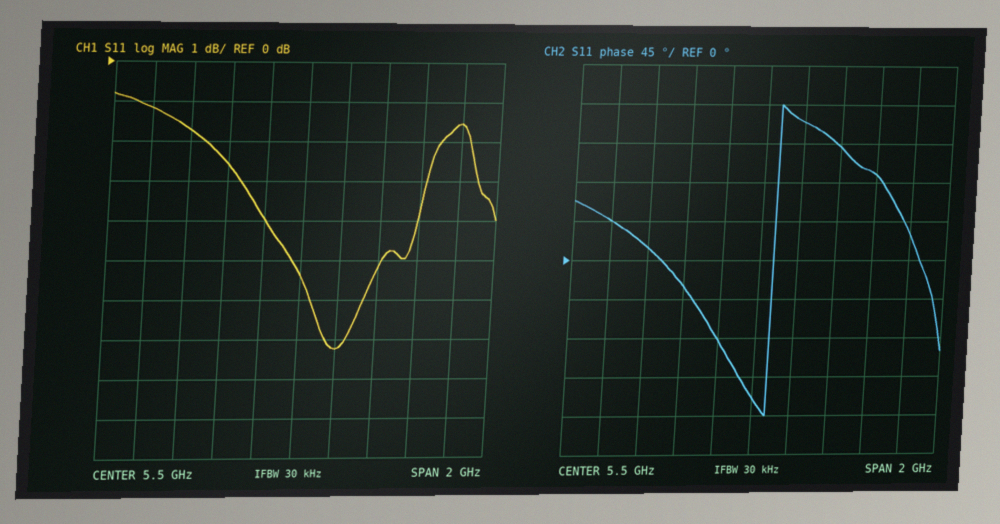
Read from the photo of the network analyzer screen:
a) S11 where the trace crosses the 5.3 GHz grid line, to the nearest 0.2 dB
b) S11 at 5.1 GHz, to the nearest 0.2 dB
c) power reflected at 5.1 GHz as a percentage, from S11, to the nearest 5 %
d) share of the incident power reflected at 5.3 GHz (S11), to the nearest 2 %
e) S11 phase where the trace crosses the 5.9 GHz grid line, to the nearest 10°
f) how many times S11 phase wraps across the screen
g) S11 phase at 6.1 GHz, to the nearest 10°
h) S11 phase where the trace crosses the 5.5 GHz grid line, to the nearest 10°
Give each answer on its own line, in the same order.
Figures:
-4.0 dB
-2.6 dB
55 %
40 %
130°
1
100°
-160°
